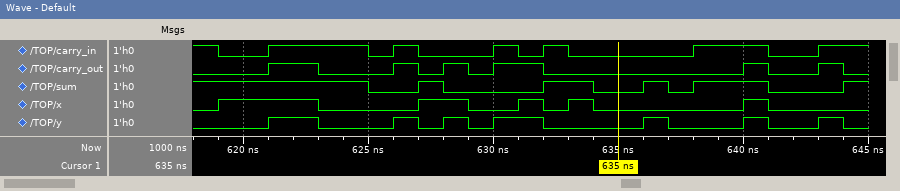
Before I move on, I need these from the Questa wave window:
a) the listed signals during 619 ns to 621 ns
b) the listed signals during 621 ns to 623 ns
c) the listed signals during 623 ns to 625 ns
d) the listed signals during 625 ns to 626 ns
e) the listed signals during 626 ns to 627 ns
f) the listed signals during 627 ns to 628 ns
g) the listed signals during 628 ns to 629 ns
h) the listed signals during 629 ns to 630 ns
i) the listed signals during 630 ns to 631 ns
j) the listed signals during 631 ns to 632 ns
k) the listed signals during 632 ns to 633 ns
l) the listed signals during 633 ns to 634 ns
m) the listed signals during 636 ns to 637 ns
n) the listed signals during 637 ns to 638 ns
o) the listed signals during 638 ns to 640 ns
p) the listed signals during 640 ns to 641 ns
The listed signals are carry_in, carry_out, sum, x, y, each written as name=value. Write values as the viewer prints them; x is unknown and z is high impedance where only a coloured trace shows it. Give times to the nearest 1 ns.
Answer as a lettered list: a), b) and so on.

a) carry_in=0, carry_out=0, sum=1, x=1, y=0
b) carry_in=1, carry_out=1, sum=1, x=1, y=1
c) carry_in=1, carry_out=0, sum=1, x=0, y=0
d) carry_in=0, carry_out=0, sum=0, x=0, y=0
e) carry_in=1, carry_out=1, sum=0, x=0, y=1
f) carry_in=0, carry_out=0, sum=1, x=1, y=0
g) carry_in=0, carry_out=1, sum=0, x=1, y=1
h) carry_in=0, carry_out=0, sum=0, x=0, y=0
i) carry_in=1, carry_out=1, sum=0, x=0, y=1
j) carry_in=0, carry_out=1, sum=0, x=1, y=1
k) carry_in=1, carry_out=0, sum=1, x=0, y=0
l) carry_in=0, carry_out=0, sum=1, x=1, y=0
m) carry_in=0, carry_out=0, sum=1, x=0, y=1
n) carry_in=0, carry_out=0, sum=0, x=0, y=0
o) carry_in=1, carry_out=0, sum=1, x=0, y=0
p) carry_in=1, carry_out=1, sum=1, x=1, y=1
